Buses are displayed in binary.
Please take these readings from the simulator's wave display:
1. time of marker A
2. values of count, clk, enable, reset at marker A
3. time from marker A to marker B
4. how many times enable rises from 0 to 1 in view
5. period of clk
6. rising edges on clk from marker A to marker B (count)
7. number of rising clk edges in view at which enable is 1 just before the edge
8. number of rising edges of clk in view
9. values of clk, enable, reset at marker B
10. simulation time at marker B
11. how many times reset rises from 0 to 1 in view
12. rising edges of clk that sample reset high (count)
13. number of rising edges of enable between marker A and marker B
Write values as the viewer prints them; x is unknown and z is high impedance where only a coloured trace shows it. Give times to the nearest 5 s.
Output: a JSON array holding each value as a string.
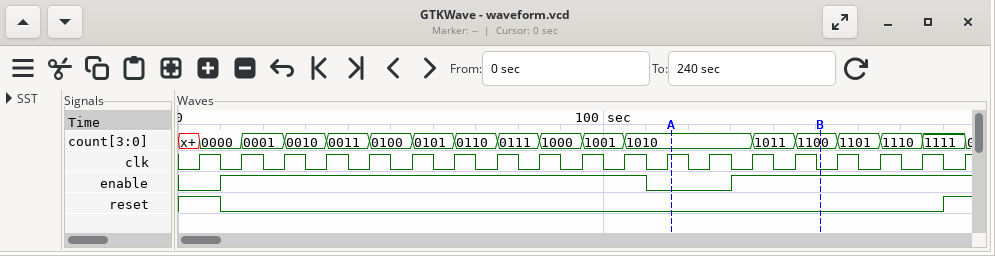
["115 s", "count=1010, clk=1, enable=0, reset=0", "35 s", "2", "10 s", "3", "16", "19", "clk=0, enable=1, reset=0", "150 s", "1", "2", "1"]
